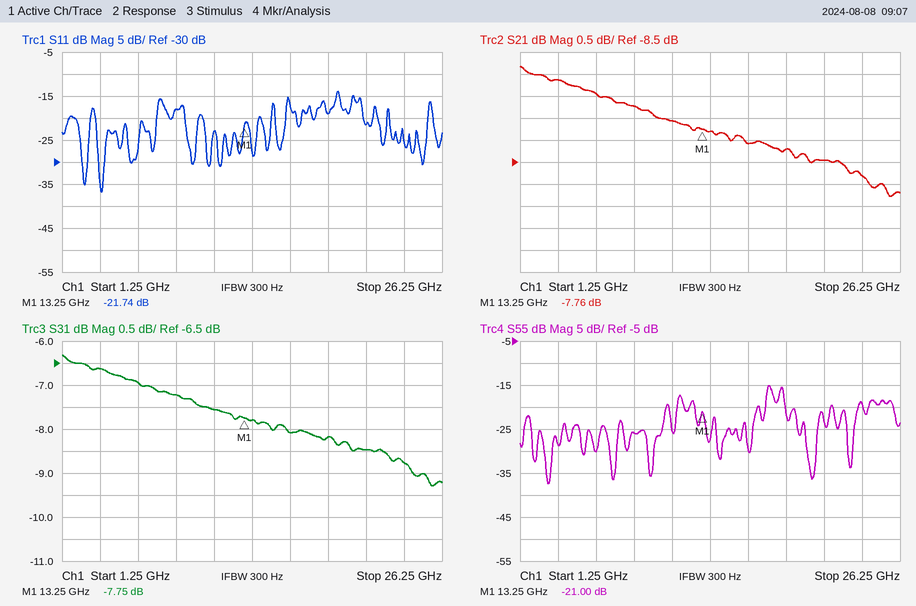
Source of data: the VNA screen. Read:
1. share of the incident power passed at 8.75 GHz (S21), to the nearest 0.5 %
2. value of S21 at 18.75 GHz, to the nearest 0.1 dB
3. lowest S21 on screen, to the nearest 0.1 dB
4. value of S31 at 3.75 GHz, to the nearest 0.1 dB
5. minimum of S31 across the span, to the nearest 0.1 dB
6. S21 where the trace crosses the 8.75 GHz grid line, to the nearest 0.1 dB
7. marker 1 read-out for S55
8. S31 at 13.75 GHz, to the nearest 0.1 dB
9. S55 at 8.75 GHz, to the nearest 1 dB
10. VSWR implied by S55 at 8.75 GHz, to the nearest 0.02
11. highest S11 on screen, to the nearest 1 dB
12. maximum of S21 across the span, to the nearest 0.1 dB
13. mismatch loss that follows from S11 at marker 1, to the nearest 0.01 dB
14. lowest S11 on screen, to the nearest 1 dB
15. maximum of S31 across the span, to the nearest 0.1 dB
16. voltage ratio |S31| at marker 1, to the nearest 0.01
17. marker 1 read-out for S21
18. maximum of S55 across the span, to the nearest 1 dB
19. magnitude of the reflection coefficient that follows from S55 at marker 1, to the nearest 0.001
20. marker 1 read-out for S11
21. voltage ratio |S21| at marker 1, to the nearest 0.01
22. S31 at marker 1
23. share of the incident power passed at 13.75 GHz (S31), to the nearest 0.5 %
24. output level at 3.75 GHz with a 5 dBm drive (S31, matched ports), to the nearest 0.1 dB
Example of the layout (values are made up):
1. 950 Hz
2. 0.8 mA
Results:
1. 19.0 %
2. -8.2 dB
3. -9.3 dB
4. -6.6 dB
5. -9.3 dB
6. -7.2 dB
7. -21.00 dB
8. -7.8 dB
9. -26 dB
10. 1.10
11. -14 dB
12. -6.3 dB
13. 0.03 dB
14. -37 dB
15. -6.3 dB
16. 0.41
17. -7.76 dB
18. -15 dB
19. 0.089
20. -21.74 dB
21. 0.41
22. -7.75 dB
23. 16.5 %
24. -1.6 dBm
